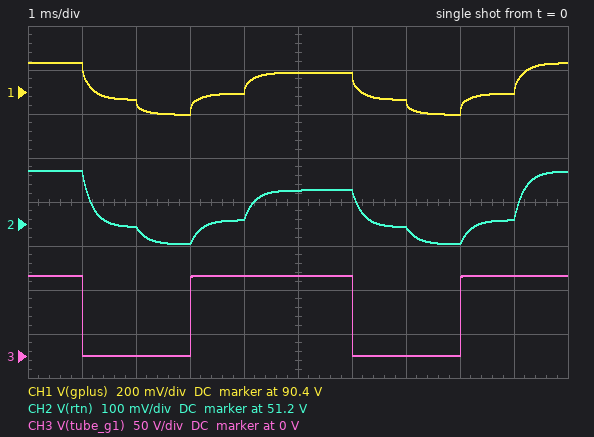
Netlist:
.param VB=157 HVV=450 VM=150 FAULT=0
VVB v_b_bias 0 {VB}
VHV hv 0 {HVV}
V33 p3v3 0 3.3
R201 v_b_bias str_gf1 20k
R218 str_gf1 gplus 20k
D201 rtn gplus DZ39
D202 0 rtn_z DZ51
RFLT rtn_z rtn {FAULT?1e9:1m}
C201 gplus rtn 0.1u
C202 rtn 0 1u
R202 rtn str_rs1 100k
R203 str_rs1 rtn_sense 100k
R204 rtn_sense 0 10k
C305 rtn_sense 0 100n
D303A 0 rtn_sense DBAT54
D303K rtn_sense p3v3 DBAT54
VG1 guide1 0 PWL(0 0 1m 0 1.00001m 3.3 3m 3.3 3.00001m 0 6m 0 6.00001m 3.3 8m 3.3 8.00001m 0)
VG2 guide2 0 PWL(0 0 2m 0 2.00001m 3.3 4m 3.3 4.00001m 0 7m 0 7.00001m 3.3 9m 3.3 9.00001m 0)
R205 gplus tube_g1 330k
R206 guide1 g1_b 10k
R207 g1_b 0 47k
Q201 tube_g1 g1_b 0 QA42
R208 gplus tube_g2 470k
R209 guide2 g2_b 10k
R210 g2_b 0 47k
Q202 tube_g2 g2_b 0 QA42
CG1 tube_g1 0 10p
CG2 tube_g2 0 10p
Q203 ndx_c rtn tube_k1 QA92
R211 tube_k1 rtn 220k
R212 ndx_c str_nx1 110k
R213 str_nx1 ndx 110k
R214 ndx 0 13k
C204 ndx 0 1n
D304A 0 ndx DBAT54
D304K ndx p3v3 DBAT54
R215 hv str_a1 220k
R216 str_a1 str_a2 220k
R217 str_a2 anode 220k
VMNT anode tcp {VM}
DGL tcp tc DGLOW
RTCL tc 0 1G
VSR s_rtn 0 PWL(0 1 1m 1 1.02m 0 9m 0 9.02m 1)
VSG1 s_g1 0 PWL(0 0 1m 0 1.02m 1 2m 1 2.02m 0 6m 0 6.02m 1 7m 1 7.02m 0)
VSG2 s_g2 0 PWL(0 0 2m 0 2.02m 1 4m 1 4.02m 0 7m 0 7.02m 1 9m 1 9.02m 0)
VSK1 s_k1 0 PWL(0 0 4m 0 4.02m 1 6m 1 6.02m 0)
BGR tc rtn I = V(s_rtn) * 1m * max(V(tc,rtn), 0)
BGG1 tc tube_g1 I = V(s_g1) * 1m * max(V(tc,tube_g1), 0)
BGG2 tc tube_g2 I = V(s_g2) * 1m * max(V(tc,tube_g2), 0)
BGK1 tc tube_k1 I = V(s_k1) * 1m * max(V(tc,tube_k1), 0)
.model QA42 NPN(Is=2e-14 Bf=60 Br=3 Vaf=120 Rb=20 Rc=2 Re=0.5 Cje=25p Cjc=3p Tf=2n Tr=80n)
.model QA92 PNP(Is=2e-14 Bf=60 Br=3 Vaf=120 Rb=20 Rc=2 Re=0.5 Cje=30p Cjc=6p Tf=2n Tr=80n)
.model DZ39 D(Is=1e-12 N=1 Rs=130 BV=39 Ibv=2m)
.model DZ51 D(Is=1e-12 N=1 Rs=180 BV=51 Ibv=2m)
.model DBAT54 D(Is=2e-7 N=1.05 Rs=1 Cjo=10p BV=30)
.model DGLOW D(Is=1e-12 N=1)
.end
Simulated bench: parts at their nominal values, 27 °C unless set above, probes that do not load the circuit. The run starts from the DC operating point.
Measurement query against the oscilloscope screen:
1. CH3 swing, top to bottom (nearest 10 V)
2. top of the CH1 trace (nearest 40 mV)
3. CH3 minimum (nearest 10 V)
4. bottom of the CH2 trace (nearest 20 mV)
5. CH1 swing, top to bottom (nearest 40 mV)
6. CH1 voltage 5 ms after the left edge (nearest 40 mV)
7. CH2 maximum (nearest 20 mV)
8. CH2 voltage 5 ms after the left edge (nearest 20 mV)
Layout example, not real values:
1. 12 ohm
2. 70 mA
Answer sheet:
1. 90 V
2. 90.52 V
3. 0 V
4. 51.16 V
5. 240 mV
6. 90.48 V
7. 51.32 V
8. 51.28 V
